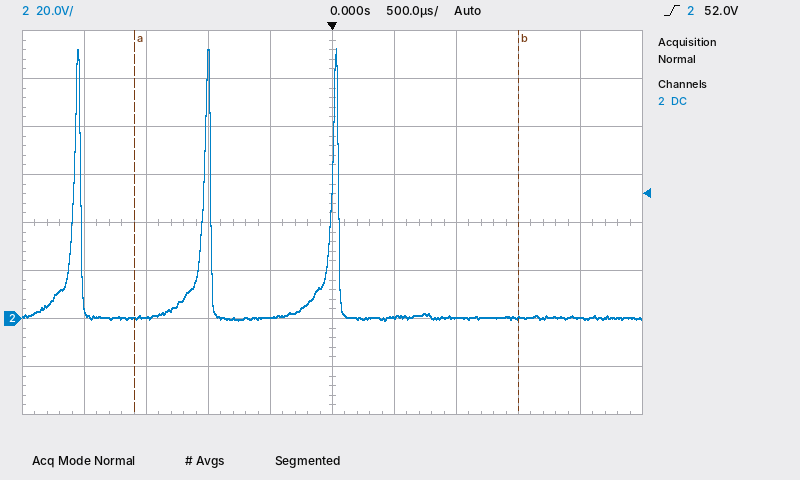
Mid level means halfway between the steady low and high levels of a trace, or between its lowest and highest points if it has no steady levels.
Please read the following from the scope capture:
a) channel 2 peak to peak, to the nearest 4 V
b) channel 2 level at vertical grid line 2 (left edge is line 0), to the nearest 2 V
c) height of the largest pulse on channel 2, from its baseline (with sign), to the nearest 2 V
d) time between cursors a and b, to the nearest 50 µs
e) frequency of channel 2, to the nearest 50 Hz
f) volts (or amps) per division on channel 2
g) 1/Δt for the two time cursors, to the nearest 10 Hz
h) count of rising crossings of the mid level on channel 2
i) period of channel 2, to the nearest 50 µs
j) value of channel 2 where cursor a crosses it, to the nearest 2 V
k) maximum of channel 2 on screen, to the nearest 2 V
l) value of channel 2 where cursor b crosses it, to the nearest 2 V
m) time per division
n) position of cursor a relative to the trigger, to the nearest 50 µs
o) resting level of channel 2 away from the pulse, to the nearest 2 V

112 V
0 V
+112 V
3.10 ms
950 Hz
20 V
320 Hz
3
1.05 ms
0 V
112 V
0 V
500 µs
-1.60 ms
0 V
